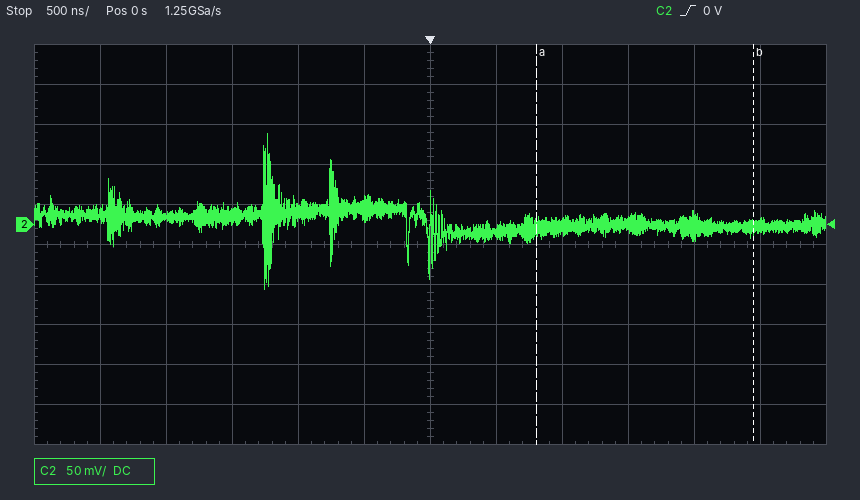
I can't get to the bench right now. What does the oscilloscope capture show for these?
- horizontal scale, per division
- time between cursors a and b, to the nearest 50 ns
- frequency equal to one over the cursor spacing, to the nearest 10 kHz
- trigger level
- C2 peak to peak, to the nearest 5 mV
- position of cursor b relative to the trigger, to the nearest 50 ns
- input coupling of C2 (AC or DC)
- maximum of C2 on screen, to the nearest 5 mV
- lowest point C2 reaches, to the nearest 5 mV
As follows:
500 ns
1.65 µs
610 kHz
0 V
195 mV
+2.45 µs
DC
115 mV
-80 mV
